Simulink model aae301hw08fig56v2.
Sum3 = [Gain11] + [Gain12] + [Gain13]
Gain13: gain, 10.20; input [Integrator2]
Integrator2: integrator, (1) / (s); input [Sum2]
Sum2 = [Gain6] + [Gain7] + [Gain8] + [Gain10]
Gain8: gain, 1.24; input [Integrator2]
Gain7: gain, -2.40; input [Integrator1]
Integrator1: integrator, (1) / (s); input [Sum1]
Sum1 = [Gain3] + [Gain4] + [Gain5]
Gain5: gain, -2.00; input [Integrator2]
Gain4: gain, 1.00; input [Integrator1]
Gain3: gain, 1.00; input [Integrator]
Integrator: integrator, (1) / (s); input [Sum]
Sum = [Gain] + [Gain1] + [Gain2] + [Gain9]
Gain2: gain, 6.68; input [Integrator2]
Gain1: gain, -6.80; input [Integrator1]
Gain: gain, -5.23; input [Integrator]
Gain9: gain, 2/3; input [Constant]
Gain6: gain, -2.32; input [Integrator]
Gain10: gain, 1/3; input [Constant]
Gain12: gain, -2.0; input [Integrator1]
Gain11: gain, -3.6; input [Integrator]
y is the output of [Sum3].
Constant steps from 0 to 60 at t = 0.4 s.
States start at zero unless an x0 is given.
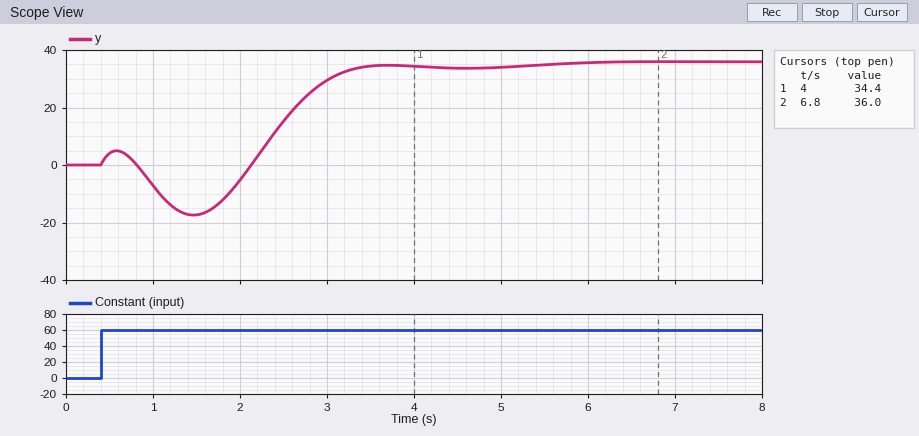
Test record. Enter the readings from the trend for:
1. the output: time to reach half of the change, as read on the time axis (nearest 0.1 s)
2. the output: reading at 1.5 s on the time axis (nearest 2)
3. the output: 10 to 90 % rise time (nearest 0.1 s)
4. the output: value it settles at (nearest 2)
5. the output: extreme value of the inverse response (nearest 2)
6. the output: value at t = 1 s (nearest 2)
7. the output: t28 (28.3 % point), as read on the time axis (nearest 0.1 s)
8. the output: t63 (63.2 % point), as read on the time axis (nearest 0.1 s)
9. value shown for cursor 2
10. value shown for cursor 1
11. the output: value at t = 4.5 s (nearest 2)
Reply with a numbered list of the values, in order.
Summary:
1. 2.6 s
2. -18
3. 2.7 s
4. 36
5. -18
6. -8
7. 2.4 s
8. 2.7 s
9. 36.0
10. 34.4
11. 34
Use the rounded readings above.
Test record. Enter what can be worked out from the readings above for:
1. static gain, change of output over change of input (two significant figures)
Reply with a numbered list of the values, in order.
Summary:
1. 0.60
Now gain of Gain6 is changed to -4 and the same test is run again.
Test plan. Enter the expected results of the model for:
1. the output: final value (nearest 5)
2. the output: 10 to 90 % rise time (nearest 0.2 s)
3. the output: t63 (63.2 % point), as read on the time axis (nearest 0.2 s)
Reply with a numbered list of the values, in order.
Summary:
1. 35
2. 1.8 s
3. 1.8 s
